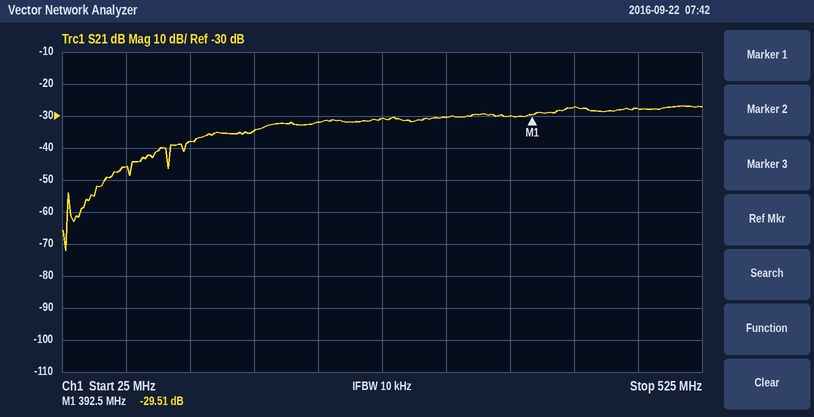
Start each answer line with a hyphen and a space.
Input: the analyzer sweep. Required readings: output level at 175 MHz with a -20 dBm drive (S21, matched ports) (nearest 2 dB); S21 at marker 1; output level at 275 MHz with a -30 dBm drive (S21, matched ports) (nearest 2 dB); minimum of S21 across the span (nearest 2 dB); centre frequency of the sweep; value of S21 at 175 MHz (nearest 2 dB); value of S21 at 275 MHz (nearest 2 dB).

- -54 dBm
- -29.51 dB
- -60 dBm
- -72 dB
- 275 MHz
- -34 dB
- -30 dB
